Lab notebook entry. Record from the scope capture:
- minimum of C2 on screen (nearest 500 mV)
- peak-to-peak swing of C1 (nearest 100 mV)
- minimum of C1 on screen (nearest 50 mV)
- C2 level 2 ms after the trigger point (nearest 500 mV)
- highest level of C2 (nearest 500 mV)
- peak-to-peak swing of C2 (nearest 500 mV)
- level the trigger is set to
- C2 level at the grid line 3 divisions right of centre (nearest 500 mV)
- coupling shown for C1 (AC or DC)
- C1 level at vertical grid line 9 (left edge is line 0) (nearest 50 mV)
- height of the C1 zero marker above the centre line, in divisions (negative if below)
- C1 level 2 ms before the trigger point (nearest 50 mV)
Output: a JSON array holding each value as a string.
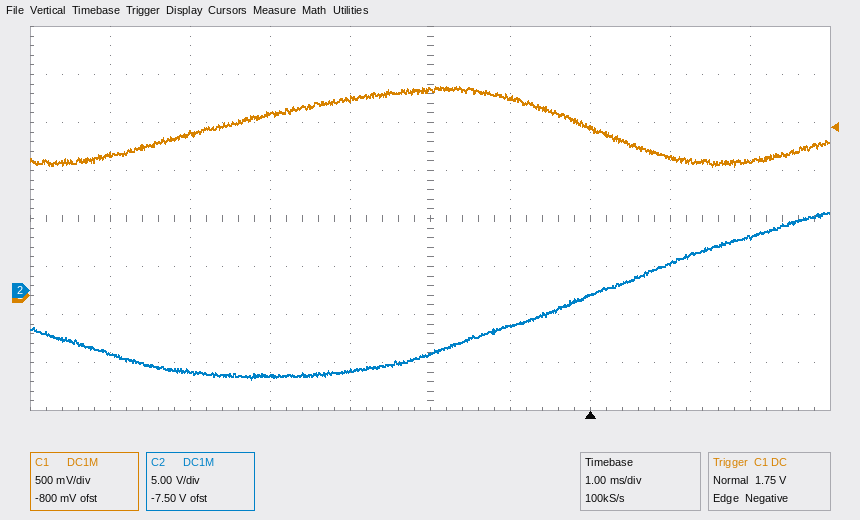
["-9.5 V", "800 mV", "1.35 V", "5.5 V", "8.0 V", "17.5 V", "1.75 V", "3.0 V", "DC", "1.40 V", "-1.6 div", "2.15 V"]
